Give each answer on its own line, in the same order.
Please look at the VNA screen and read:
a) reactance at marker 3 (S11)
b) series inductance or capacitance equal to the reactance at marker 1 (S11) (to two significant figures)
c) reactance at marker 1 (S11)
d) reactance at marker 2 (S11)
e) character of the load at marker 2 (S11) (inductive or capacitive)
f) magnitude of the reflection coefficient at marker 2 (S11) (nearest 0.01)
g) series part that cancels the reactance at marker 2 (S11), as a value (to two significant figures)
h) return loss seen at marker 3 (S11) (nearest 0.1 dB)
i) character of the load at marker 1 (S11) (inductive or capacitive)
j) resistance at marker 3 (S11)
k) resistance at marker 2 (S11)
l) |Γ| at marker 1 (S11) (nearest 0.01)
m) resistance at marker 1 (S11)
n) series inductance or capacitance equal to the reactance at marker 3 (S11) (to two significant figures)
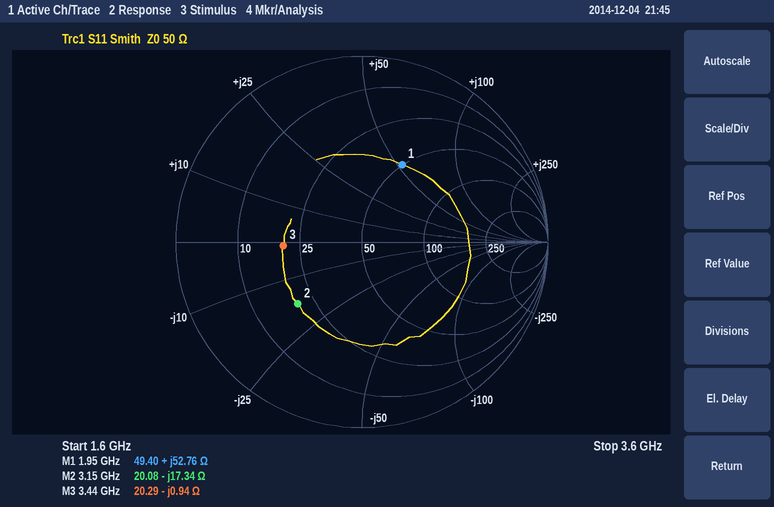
-0.94 Ω
4.3 nH
+52.76 Ω
-17.34 Ω
capacitive
0.48
880 pH
7.5 dB
inductive
20.29 Ω
20.08 Ω
0.47
49.40 Ω
49 pF
